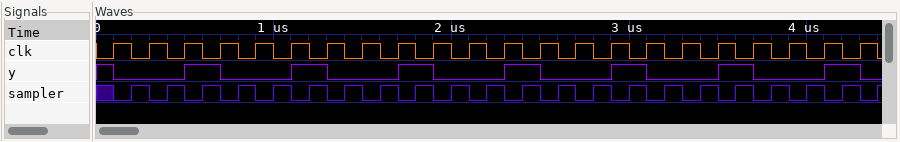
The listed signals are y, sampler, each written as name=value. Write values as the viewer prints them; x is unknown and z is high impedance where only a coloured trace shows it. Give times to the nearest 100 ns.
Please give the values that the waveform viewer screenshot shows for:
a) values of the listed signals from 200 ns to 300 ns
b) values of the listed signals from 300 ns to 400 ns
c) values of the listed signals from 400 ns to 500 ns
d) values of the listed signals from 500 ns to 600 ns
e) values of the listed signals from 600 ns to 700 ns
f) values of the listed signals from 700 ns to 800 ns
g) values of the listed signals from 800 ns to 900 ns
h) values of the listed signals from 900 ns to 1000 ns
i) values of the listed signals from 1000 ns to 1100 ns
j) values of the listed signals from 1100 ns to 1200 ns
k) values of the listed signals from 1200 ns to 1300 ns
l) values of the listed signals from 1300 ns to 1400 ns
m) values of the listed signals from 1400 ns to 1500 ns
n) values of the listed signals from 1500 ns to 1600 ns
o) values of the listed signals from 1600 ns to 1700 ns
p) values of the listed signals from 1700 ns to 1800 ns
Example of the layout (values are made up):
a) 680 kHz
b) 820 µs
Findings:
a) y=0, sampler=1
b) y=0, sampler=0
c) y=0, sampler=1
d) y=1, sampler=0
e) y=1, sampler=1
f) y=0, sampler=0
g) y=0, sampler=1
h) y=0, sampler=0
i) y=0, sampler=1
j) y=1, sampler=0
k) y=1, sampler=1
l) y=0, sampler=0
m) y=0, sampler=1
n) y=0, sampler=0
o) y=0, sampler=1
p) y=1, sampler=0
